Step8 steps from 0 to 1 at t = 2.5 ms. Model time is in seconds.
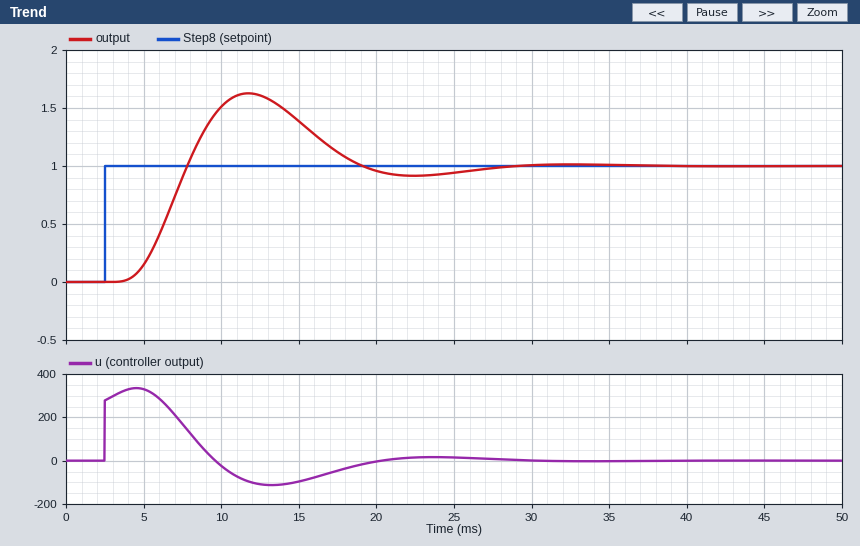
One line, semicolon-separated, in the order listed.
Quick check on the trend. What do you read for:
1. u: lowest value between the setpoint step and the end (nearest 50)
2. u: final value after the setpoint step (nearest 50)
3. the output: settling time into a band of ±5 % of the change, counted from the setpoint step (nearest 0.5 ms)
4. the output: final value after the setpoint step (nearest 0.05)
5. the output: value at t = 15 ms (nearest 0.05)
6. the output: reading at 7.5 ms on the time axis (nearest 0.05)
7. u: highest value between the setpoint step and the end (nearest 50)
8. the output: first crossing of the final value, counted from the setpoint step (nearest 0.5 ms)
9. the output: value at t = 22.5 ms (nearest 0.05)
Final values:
-100; 0; 23.0 ms; 1.00; 1.40; 0.90; 350; 5.5 ms; 0.90
